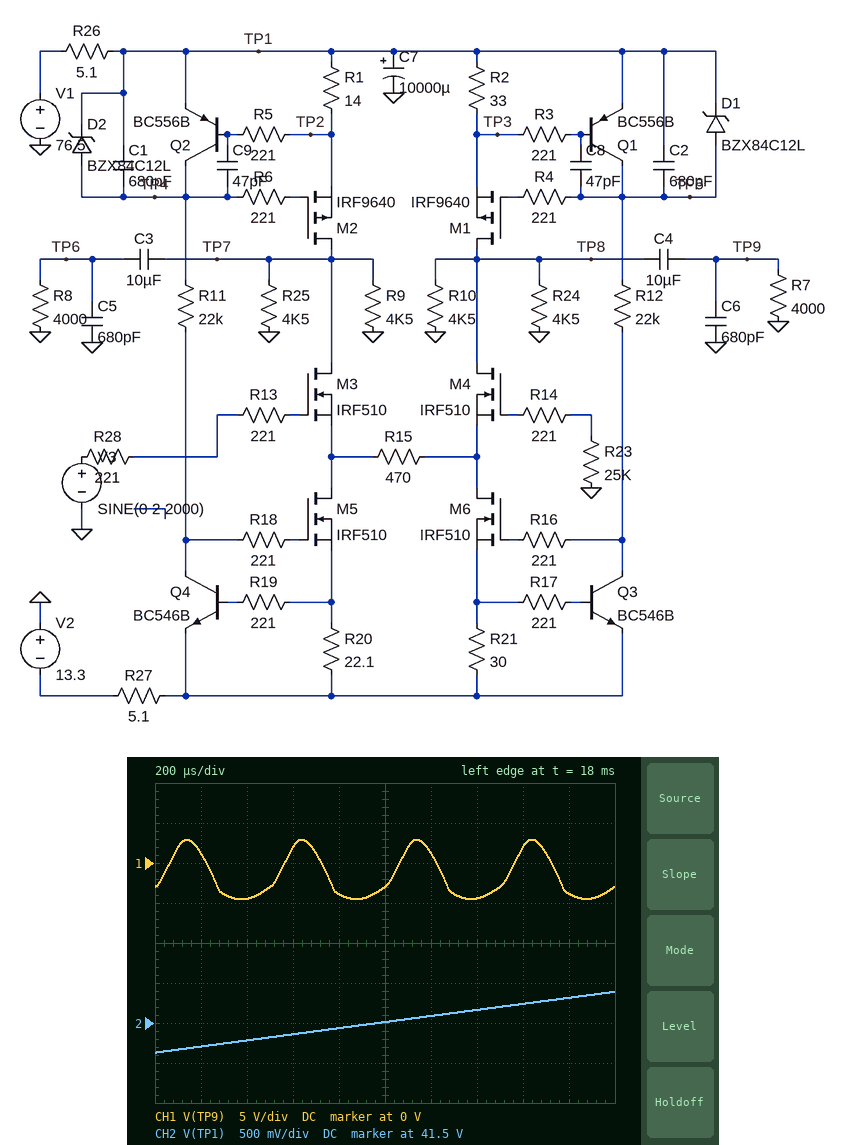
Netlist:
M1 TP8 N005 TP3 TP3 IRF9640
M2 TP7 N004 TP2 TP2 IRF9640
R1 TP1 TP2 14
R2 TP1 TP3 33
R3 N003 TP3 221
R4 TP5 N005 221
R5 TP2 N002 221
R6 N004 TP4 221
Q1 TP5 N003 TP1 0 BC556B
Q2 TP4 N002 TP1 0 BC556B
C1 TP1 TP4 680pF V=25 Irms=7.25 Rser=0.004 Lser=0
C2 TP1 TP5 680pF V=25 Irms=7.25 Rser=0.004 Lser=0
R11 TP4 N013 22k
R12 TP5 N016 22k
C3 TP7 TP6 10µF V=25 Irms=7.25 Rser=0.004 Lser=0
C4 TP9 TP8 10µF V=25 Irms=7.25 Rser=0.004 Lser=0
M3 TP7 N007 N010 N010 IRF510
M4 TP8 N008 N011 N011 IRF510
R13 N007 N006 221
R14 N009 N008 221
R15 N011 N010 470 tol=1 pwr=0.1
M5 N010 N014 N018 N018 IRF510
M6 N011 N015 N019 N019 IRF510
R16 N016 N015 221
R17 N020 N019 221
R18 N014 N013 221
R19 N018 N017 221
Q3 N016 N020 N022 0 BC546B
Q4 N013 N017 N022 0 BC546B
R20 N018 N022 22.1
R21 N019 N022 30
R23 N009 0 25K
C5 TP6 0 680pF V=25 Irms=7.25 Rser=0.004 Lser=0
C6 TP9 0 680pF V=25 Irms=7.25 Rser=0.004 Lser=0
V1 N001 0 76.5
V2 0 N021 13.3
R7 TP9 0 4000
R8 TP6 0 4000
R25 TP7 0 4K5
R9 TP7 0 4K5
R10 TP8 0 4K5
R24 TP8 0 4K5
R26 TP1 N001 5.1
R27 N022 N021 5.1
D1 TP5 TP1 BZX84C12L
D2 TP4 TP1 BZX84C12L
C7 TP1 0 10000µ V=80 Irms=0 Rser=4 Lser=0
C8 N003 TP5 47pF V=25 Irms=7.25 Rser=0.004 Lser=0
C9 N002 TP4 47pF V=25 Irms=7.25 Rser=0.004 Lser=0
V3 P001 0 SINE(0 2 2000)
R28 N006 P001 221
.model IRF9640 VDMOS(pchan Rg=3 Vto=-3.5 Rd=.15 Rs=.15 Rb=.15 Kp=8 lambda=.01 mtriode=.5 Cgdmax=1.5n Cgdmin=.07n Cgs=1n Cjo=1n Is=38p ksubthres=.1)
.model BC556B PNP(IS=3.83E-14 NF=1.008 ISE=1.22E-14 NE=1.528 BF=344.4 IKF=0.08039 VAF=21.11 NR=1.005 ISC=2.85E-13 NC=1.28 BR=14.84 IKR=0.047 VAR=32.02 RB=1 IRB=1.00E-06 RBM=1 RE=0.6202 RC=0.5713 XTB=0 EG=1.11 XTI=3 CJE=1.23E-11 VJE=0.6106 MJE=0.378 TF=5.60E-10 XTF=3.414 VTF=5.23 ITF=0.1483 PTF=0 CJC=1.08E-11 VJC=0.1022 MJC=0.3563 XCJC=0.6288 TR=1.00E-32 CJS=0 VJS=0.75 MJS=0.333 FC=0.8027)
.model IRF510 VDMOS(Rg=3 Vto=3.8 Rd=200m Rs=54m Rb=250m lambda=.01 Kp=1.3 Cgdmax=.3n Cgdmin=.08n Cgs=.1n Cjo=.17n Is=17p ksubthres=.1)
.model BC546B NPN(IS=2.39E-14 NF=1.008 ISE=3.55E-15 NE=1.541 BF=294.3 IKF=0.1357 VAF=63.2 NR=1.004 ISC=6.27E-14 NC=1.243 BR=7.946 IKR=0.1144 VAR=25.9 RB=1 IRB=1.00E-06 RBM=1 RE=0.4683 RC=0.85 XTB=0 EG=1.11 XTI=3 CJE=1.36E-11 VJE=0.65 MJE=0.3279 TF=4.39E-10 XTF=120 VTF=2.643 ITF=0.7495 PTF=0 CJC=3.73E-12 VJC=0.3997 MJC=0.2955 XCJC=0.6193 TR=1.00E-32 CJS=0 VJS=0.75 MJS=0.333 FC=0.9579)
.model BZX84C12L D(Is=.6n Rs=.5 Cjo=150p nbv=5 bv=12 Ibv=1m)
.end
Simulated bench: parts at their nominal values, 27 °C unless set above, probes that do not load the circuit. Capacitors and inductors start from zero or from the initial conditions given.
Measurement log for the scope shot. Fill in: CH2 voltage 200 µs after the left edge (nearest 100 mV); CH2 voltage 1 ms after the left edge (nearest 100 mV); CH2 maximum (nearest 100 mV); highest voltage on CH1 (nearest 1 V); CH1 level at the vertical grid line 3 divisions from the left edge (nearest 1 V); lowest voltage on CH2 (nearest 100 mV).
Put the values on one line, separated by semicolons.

41.2 V; 41.5 V; 41.9 V; 3 V; 2 V; 41.1 V
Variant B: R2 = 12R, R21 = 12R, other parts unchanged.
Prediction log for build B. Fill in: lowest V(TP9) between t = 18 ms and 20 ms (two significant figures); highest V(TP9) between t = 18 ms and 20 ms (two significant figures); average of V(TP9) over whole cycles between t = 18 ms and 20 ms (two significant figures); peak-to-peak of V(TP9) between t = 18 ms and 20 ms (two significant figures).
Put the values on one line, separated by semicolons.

-4.6 V; 4.7 V; -630 mV; 9.3 V
